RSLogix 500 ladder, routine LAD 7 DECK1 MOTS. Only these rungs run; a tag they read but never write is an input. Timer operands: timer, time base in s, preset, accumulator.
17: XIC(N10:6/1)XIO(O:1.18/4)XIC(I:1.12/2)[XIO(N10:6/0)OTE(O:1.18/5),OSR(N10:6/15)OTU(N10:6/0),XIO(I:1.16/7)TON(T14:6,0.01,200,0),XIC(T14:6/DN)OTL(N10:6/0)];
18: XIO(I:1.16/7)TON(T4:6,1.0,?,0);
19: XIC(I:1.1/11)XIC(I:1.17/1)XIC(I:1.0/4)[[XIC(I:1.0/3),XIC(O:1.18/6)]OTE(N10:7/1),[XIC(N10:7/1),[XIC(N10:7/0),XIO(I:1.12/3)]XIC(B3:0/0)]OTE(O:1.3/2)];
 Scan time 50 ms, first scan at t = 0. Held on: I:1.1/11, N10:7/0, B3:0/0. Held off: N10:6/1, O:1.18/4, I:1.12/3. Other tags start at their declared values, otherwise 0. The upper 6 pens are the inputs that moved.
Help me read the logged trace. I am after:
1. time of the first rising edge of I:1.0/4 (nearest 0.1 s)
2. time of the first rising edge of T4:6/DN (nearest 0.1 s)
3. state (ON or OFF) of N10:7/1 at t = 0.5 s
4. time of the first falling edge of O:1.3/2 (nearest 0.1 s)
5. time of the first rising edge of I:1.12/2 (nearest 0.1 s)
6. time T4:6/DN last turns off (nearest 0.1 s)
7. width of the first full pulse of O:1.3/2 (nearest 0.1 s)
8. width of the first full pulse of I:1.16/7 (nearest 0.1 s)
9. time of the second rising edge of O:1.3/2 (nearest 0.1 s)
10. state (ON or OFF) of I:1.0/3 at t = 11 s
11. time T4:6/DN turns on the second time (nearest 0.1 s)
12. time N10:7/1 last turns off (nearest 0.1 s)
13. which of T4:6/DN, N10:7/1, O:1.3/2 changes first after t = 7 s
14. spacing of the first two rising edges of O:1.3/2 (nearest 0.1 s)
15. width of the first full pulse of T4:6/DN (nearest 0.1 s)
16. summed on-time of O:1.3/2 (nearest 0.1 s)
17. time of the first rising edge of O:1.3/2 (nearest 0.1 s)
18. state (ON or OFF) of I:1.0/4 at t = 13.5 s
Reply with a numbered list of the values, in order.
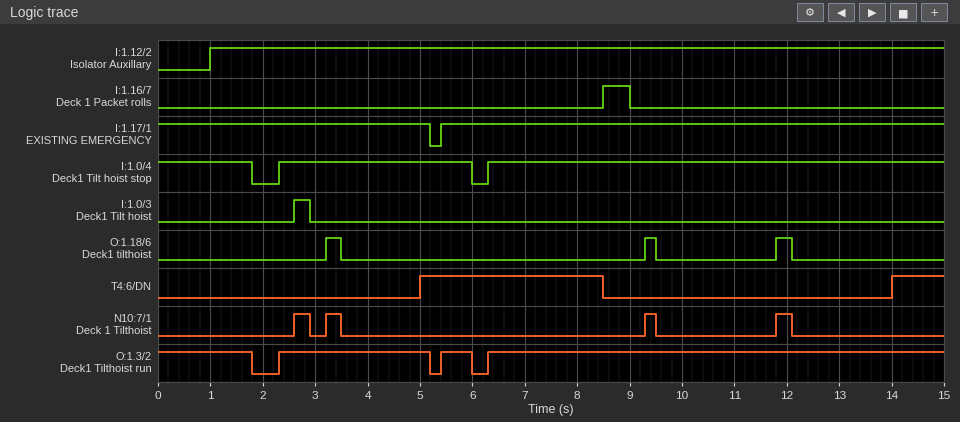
1. 2.3 s
2. 5.0 s
3. OFF
4. 1.8 s
5. 1.0 s
6. 8.5 s
7. 2.9 s
8. 0.5 s
9. 5.4 s
10. OFF
11. 14.0 s
12. 12.1 s
13. T4:6/DN
14. 3.1 s
15. 3.5 s
16. 14.0 s
17. 2.3 s
18. ON
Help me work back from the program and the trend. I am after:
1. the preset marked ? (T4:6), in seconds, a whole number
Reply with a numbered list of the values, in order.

1. 5 s
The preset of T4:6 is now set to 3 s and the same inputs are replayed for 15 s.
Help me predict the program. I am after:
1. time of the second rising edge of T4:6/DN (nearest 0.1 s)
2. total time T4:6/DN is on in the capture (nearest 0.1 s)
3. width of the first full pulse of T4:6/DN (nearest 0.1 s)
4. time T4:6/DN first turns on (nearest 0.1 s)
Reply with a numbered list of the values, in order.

1. 12.0 s
2. 8.5 s
3. 5.5 s
4. 3.0 s
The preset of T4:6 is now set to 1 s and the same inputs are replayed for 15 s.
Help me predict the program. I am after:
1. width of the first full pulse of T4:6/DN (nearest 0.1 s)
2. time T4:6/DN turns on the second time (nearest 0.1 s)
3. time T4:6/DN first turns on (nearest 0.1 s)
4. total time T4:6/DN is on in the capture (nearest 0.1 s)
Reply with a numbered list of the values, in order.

1. 7.5 s
2. 10.0 s
3. 1.0 s
4. 12.5 s
